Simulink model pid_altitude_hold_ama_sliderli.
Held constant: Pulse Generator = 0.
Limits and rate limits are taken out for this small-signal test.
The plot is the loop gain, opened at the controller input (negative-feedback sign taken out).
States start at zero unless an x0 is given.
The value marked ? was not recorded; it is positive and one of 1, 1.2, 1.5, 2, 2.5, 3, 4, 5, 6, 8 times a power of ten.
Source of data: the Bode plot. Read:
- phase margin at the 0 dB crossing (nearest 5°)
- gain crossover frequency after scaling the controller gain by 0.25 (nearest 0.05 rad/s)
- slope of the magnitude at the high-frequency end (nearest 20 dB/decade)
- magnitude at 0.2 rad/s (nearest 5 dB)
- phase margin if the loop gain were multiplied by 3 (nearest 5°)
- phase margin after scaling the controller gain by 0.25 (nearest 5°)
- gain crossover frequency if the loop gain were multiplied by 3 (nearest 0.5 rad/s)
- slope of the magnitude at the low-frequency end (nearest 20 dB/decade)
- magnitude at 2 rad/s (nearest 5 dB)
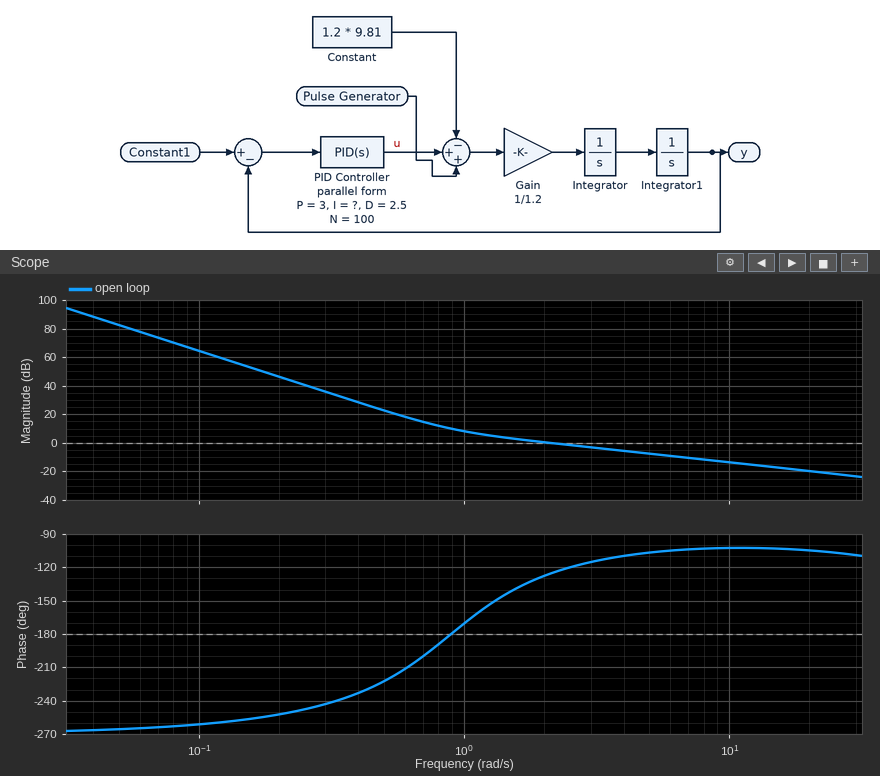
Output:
55°
0.80 rad/s
-20 dB/decade
45 dB
75°
-10°
6.5 rad/s
-60 dB/decade
0 dB
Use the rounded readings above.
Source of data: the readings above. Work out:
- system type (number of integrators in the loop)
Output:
3
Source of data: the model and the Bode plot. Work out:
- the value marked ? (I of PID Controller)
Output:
2
